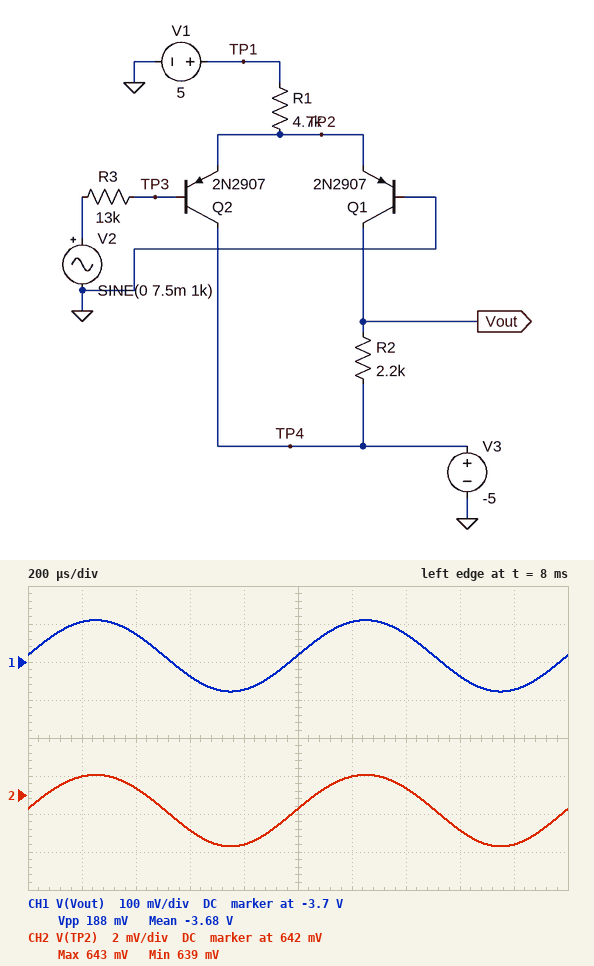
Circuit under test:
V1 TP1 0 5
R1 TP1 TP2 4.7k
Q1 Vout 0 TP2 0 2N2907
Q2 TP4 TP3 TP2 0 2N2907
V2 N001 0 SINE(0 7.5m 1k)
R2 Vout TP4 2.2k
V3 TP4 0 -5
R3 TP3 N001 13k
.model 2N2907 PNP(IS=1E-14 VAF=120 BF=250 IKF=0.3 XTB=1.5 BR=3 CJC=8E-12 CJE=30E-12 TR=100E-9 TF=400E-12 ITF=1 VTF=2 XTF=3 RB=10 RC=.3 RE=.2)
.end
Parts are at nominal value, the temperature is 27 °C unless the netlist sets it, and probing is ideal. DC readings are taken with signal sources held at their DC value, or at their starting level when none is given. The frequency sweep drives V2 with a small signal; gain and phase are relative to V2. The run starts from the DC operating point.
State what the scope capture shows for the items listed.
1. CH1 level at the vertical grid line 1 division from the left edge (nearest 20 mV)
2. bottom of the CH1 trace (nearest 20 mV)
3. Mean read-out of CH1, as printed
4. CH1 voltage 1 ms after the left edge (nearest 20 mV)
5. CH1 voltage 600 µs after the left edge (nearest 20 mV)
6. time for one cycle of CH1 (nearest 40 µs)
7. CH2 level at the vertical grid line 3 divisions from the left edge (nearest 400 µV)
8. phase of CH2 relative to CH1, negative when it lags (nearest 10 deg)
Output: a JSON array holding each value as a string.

["-3.60 V", "-3.78 V", "-3.68 V", "-3.68 V", "-3.74 V", "1.00 ms", "640.0 mV", "0 deg"]
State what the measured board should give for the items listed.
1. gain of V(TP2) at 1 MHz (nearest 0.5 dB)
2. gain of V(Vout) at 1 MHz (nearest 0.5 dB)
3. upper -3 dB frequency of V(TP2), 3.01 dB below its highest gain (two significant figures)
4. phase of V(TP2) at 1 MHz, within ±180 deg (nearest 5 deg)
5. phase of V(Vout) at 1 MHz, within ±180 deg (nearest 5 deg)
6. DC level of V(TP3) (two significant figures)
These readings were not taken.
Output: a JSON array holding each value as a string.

["-19.5 dB", "14.5 dB", "460 kHz", "-65 deg", "-70 deg", "16 mV"]
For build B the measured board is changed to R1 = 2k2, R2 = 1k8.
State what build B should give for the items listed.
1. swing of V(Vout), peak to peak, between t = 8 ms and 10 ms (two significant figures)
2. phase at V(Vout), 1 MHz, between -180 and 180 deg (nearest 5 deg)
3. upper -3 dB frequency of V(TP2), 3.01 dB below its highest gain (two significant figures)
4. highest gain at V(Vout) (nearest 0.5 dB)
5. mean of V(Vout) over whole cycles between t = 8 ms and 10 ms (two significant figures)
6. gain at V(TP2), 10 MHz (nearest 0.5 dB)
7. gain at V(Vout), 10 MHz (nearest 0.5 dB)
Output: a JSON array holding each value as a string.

["230 mV", "-65 deg", "490 kHz", "23.5 dB", "-2.4 V", "-41.0 dB", "-4.0 dB"]
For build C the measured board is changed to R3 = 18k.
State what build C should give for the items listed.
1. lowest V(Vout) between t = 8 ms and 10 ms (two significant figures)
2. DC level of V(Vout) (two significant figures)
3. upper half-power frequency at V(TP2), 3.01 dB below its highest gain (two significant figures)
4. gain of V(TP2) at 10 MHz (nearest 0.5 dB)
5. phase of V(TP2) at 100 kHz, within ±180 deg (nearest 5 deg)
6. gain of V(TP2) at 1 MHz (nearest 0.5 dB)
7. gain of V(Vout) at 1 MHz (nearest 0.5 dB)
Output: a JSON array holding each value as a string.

["-3.7 V", "-3.6 V", "350 kHz", "-42.0 dB", "-15 deg", "-23.0 dB", "11.0 dB"]
